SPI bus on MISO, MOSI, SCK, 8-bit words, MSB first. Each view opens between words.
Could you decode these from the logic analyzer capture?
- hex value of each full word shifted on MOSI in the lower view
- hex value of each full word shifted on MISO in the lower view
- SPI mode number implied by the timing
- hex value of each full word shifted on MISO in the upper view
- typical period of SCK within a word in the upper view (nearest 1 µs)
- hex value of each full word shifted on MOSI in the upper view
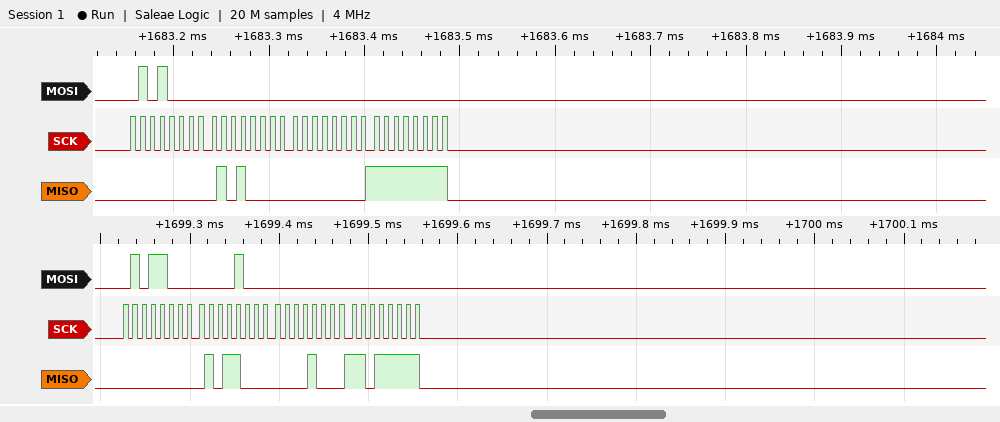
58, 08, 00, 00
00, 58, 08, DF
0
00, 50, 00, FF
10 µs
50, 00, 00, 00
